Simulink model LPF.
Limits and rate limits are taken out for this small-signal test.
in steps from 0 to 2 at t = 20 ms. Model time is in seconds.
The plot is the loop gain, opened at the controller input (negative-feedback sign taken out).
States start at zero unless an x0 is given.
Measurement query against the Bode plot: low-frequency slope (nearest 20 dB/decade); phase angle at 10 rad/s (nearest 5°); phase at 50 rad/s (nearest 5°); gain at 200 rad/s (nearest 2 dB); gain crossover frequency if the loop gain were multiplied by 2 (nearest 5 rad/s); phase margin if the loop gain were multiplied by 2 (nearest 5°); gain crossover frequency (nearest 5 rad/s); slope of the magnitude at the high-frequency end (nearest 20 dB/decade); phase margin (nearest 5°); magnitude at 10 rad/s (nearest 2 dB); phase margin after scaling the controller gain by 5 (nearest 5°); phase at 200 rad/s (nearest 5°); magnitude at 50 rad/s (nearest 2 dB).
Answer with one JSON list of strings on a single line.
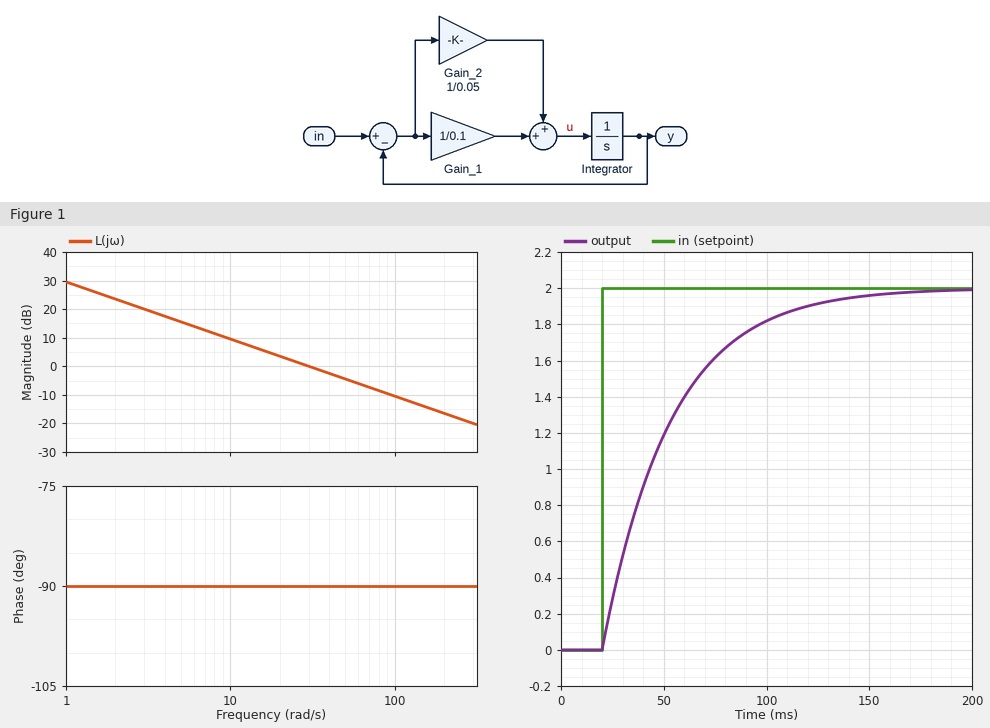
["-20 dB/decade", "-90°", "-90°", "-16 dB", "60 rad/s", "90°", "30 rad/s", "-20 dB/decade", "90°", "10 dB", "90°", "-90°", "-4 dB"]
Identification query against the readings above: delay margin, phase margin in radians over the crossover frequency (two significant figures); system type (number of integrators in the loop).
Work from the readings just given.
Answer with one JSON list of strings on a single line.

["0.052 s", "1"]
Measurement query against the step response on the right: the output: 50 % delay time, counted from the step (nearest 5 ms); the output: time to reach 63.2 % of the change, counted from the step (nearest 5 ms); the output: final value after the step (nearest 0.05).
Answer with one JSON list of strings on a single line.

["25 ms", "35 ms", "2.00"]
